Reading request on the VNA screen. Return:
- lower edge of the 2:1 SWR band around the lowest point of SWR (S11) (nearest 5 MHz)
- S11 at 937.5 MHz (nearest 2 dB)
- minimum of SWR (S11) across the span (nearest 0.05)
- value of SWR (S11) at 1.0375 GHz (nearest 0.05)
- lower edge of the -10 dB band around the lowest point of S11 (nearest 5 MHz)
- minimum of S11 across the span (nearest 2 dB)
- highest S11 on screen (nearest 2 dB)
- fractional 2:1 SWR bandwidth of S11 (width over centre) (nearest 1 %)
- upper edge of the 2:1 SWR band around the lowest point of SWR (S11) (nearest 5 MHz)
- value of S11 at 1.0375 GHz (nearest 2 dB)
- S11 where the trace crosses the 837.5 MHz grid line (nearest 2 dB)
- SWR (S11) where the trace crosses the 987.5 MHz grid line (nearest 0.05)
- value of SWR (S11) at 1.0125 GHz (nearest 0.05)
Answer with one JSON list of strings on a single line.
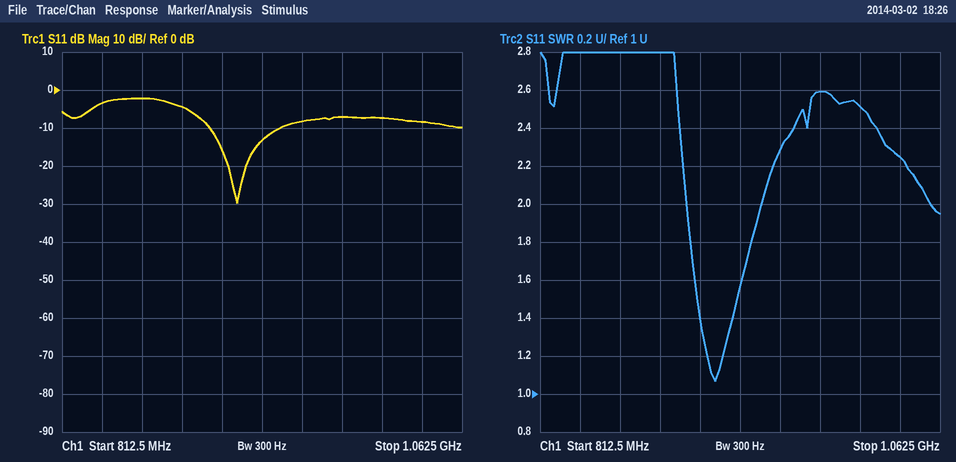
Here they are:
["905 MHz", "-14 dB", "1.05", "2.25", "905 MHz", "-30 dB", "-2 dB", "5 %", "950 MHz", "-8 dB", "-4 dB", "2.60", "2.50"]
